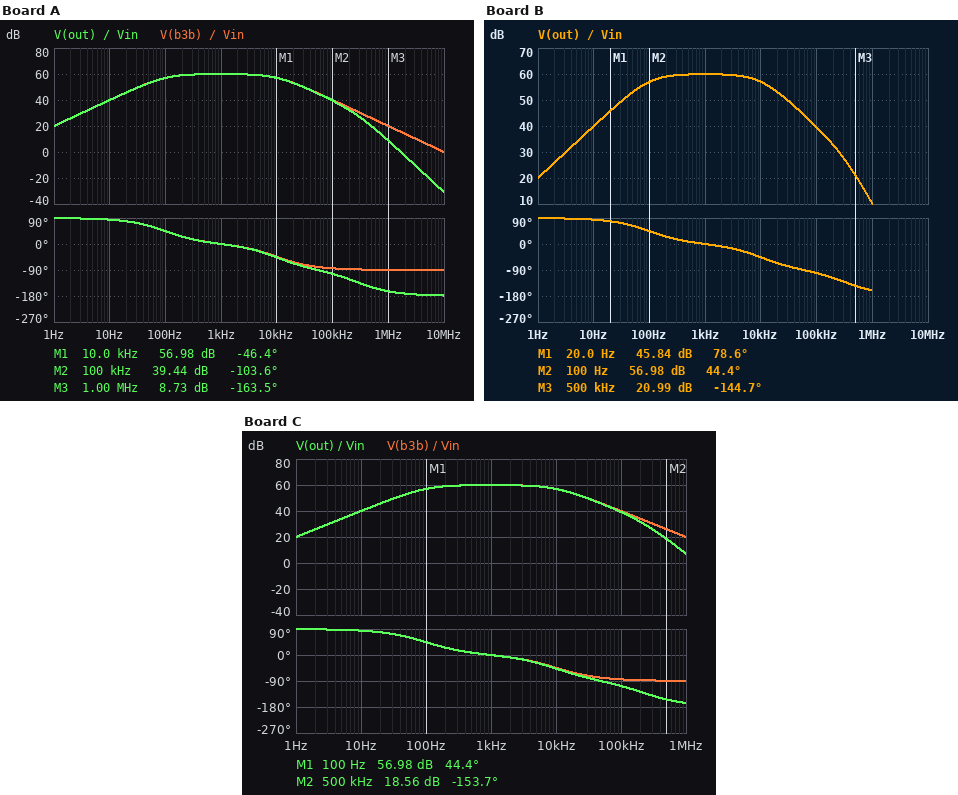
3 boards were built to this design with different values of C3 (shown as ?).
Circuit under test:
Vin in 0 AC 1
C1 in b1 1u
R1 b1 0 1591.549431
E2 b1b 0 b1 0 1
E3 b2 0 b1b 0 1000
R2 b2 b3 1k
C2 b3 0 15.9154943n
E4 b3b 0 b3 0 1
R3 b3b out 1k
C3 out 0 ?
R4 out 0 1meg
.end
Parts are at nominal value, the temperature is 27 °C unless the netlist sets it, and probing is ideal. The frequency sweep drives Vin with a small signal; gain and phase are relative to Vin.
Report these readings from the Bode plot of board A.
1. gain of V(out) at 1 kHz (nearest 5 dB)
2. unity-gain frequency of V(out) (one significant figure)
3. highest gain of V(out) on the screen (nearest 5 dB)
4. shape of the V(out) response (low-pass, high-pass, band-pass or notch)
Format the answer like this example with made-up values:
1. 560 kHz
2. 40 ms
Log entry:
1. 60 dB
2. 2 MHz
3. 60 dB
4. band-pass
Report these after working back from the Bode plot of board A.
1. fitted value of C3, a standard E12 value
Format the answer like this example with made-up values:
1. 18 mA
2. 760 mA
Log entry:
1. 560 pF
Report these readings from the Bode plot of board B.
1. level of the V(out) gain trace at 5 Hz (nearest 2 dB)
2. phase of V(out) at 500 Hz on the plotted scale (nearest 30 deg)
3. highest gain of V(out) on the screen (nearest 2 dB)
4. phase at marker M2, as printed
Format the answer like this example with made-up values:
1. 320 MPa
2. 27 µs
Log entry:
1. 34 dB
2. 0 deg
3. 60 dB
4. 44.4 deg
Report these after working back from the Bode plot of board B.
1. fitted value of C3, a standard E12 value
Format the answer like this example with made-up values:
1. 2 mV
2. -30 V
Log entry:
1. 470 pF
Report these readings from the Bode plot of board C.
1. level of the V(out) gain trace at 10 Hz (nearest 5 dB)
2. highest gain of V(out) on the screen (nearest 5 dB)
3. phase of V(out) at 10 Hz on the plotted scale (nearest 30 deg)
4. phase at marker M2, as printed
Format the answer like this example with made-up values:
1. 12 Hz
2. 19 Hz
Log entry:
1. 40 dB
2. 60 dB
3. 90 deg
4. -153.7 deg
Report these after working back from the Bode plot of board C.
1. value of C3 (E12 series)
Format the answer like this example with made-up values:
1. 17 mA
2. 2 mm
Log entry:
1. 680 pF
